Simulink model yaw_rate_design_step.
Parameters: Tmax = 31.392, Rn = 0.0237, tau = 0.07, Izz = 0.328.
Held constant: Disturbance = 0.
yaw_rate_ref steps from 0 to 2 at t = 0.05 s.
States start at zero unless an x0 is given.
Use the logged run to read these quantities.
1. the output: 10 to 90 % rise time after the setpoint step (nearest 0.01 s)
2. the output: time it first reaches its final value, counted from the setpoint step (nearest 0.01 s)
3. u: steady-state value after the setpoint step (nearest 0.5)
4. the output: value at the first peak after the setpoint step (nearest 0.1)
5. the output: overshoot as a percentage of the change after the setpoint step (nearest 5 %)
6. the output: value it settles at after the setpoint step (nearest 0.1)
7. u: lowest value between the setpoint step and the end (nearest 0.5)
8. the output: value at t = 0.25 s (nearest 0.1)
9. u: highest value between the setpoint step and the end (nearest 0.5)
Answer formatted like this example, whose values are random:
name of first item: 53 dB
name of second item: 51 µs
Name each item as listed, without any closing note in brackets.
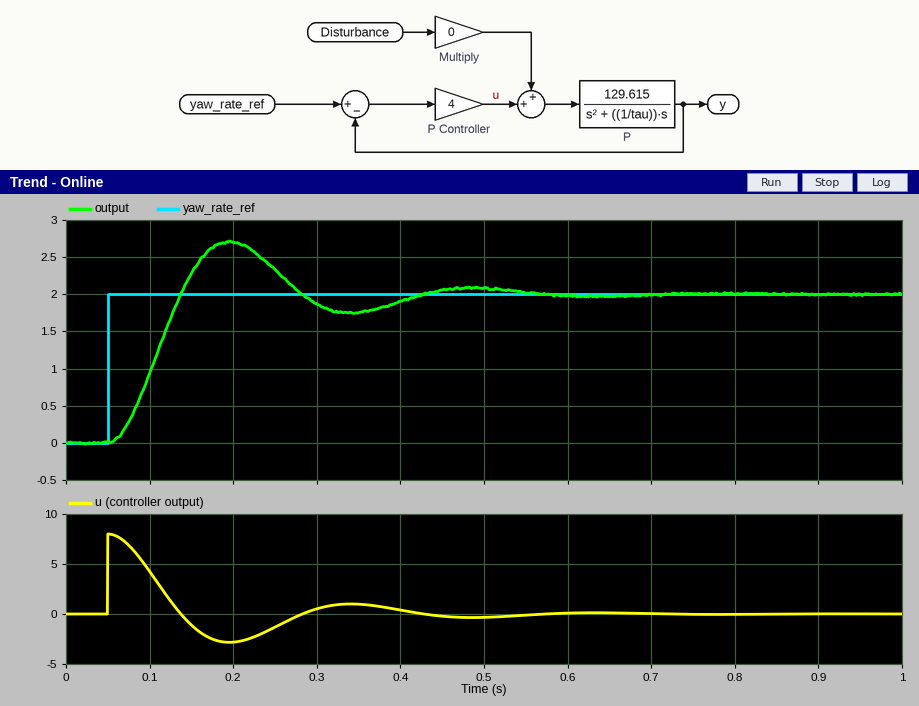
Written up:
the output: 10 to 90 % rise time after the setpoint step: 0.06 s
the output: time it first reaches its final value, counted from the setpoint step: 0.09 s
u: steady-state value after the setpoint step: 0.0
the output: value at the first peak after the setpoint step: 2.7
the output: overshoot as a percentage of the change after the setpoint step: 35 %
the output: value it settles at after the setpoint step: 2.0
u: lowest value between the setpoint step and the end: -3.0
the output: value at t = 0.25 s: 2.3
u: highest value between the setpoint step and the end: 8.0
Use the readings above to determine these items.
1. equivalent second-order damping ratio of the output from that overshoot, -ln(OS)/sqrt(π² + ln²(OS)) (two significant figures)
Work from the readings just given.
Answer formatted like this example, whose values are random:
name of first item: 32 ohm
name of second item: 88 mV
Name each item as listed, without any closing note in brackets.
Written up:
equivalent second-order damping ratio of the output from that overshoot, -ln(OS)/sqrt(π² + ln²(OS)): 0.32
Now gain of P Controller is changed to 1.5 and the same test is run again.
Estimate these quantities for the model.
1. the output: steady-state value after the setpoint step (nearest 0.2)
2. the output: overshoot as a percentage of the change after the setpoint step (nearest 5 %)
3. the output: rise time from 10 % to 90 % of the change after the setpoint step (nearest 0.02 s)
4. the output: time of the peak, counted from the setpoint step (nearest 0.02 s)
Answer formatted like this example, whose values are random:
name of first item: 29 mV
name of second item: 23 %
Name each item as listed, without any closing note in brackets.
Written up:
the output: steady-state value after the setpoint step: 2.0
the output: overshoot as a percentage of the change after the setpoint step: 15 %
the output: rise time from 10 % to 90 % of the change after the setpoint step: 0.12 s
the output: time of the peak, counted from the setpoint step: 0.26 s
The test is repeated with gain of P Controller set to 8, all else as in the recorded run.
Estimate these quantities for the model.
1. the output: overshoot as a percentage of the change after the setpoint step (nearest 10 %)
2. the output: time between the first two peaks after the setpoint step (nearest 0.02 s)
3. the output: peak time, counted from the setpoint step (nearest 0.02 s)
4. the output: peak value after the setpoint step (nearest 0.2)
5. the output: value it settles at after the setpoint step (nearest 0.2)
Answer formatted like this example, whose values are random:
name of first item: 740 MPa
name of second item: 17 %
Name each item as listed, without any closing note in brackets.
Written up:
the output: overshoot as a percentage of the change after the setpoint step: 50 %
the output: time between the first two peaks after the setpoint step: 0.20 s
the output: peak time, counted from the setpoint step: 0.10 s
the output: peak value after the setpoint step: 3.0
the output: value it settles at after the setpoint step: 2.0
